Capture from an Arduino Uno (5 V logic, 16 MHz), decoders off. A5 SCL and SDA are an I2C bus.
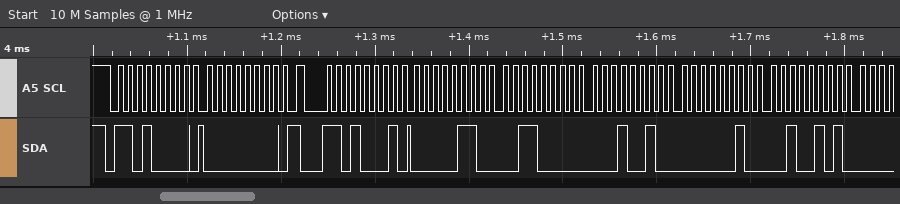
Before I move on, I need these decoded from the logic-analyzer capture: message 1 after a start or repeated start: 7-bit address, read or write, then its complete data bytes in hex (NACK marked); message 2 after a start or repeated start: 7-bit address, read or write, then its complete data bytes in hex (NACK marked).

0x68 write: 00
0x68 read: 06 30 12 02 25
